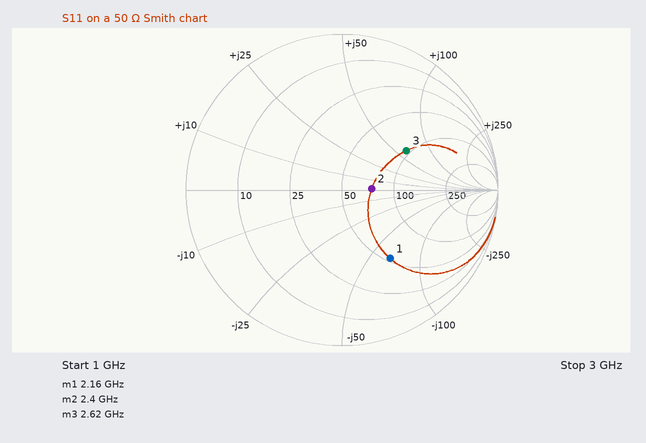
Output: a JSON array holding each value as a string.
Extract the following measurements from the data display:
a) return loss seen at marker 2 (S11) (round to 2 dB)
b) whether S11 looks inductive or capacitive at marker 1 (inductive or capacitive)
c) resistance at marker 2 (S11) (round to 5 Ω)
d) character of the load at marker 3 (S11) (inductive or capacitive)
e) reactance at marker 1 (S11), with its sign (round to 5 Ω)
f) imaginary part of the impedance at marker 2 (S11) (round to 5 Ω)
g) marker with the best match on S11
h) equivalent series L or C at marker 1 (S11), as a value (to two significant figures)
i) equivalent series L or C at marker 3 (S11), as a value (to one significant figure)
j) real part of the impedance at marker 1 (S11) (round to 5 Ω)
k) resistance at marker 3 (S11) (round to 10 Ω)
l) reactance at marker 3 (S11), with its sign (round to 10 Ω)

["14 dB", "capacitive", "75 Ω", "inductive", "-65 Ω", "0 Ω", "marker 2", "1.1 pF", "4 nH", "55 Ω", "90 Ω", "+60 Ω"]
